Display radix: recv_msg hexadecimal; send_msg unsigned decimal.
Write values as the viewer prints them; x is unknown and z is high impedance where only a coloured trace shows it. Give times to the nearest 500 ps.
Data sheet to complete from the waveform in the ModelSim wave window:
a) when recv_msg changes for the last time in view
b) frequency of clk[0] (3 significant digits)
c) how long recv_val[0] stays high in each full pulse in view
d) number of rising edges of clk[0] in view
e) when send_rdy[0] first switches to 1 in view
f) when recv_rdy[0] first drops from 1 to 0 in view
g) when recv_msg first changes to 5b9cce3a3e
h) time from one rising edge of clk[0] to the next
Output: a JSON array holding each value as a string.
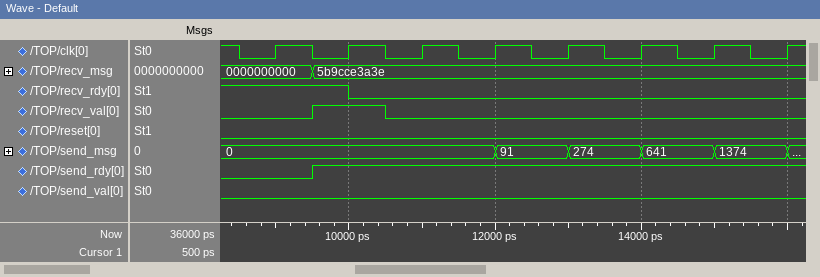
["9500 ps", "1.00 GHz", "1000 ps", "8", "9500 ps", "10000 ps", "9500 ps", "1000 ps"]
